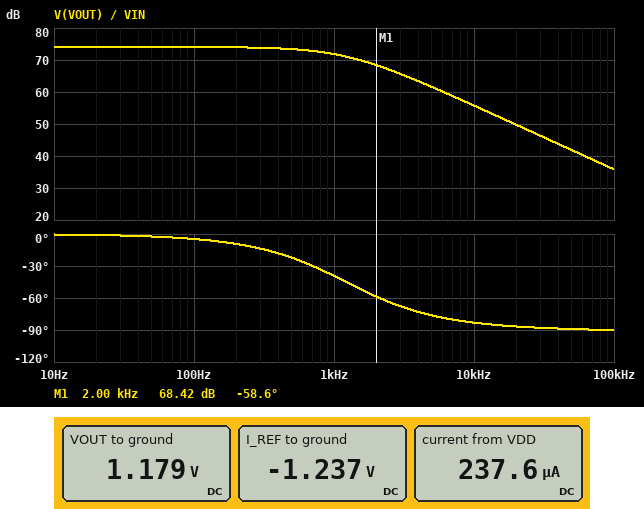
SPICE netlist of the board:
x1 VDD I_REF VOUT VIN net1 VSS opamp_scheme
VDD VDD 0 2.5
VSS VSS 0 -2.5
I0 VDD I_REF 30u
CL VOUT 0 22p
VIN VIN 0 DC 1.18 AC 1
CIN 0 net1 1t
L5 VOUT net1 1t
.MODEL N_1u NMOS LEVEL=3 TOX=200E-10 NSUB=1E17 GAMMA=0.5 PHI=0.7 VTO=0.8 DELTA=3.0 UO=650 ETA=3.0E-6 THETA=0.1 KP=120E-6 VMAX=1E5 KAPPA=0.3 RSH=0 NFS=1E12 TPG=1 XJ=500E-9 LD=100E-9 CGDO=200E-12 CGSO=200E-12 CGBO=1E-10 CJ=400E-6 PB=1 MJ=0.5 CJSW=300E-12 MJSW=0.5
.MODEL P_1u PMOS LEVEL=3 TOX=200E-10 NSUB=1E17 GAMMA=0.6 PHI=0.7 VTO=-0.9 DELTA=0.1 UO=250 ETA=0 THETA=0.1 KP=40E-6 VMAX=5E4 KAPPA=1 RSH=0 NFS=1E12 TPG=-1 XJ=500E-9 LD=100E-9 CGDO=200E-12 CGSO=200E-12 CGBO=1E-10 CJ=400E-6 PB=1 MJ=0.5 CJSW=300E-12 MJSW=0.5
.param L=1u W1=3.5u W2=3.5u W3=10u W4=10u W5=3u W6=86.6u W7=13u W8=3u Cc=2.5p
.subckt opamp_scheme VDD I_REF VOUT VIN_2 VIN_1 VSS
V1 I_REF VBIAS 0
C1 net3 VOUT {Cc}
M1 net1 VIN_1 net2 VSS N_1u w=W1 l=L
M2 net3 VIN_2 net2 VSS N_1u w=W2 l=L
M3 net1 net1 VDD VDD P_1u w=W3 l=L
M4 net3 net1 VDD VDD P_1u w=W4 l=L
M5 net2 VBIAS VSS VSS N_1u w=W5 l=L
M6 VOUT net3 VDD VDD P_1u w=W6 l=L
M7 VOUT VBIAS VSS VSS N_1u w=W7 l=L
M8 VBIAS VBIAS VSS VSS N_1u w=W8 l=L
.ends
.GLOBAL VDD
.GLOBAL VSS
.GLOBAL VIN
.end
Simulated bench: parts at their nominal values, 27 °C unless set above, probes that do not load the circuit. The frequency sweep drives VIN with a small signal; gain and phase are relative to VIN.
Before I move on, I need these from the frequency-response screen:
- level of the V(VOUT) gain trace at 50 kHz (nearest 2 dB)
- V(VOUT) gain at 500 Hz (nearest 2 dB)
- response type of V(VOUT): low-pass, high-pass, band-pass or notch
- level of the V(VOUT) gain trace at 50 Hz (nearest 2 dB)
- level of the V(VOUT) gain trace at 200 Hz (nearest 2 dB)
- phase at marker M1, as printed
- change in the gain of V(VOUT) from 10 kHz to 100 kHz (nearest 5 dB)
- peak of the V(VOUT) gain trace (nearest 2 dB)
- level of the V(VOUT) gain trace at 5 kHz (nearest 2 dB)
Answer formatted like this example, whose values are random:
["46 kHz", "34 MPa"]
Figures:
["42 dB", "74 dB", "low-pass", "74 dB", "74 dB", "-58.6 deg", "-20 dB", "74 dB", "62 dB"]
